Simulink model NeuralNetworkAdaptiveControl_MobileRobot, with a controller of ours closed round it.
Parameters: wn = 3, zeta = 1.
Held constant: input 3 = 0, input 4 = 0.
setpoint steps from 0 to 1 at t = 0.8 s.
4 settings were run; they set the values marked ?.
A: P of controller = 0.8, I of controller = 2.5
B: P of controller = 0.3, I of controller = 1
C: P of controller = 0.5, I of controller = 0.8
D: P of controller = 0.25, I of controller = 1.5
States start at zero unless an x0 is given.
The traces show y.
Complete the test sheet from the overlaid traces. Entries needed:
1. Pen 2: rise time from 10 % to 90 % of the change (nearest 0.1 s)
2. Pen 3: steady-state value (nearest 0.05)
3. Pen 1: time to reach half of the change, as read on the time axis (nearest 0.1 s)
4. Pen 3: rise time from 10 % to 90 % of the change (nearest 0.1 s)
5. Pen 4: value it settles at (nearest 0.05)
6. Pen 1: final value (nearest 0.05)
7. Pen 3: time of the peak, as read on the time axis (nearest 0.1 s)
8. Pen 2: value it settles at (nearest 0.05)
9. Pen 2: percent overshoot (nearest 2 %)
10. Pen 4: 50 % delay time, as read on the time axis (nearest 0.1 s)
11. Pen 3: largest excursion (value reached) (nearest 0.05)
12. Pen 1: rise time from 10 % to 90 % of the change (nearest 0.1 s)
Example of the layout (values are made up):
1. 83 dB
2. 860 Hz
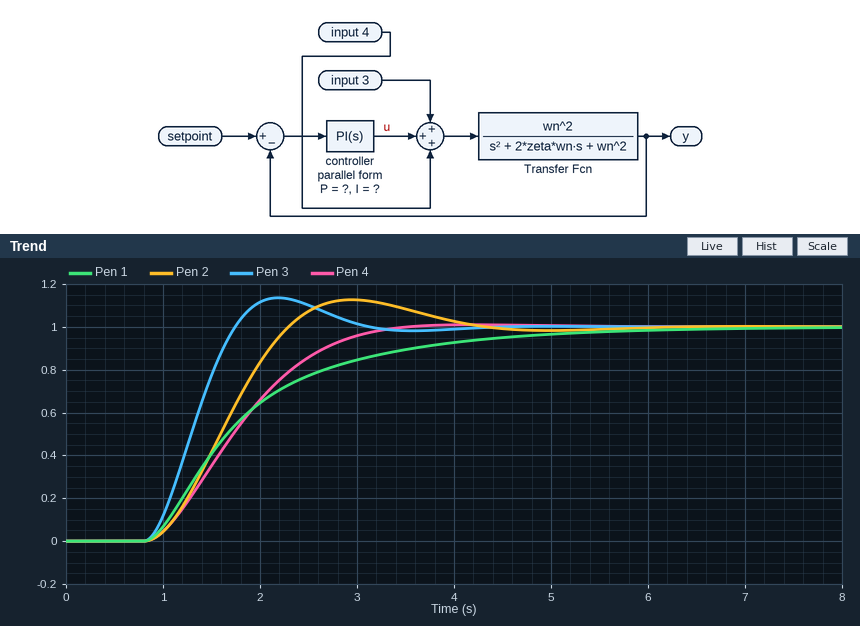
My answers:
1. 1.0 s
2. 1.00
3. 1.7 s
4. 0.6 s
5. 1.00
6. 1.00
7. 2.2 s
8. 1.00
9. 12 %
10. 1.7 s
11. 1.15
12. 2.5 s
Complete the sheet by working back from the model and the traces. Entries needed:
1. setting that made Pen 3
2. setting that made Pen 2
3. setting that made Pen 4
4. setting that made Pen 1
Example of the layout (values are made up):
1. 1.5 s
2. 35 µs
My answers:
1. A
2. D
3. B
4. C
